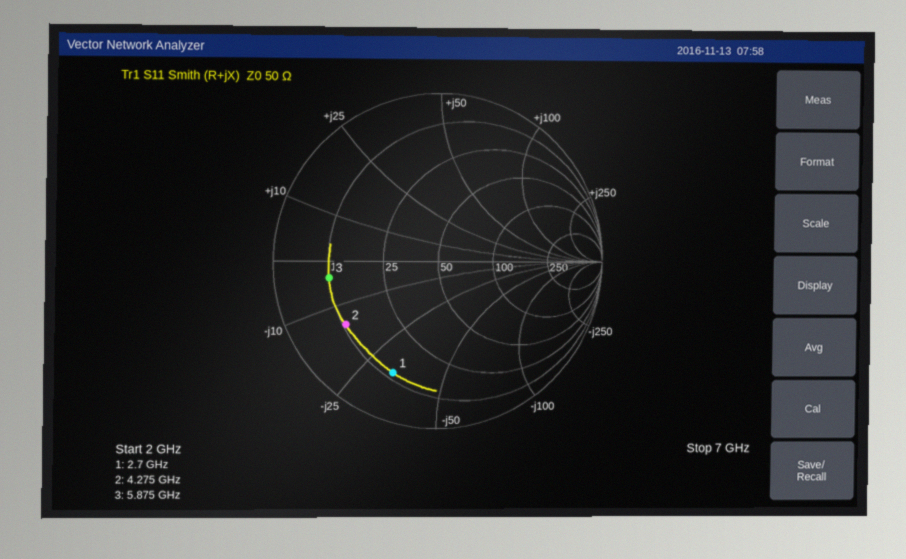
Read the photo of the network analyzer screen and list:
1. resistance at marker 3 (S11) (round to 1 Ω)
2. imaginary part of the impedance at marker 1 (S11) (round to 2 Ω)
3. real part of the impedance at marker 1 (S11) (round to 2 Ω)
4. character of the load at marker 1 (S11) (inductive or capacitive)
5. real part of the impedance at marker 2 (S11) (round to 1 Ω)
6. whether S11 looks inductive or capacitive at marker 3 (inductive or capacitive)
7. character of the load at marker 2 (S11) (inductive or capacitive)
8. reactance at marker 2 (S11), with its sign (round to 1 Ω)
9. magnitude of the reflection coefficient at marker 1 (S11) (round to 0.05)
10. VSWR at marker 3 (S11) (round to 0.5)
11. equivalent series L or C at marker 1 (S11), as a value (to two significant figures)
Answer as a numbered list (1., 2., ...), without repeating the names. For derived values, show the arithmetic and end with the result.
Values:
1. 10 Ω
2. -32 Ω
3. 12 Ω
4. capacitive
5. 11 Ω
6. capacitive
7. capacitive
8. -15 Ω
9. 0.70
10. 5.0
11. C = 1/(2π × 2.7 GHz × 32 Ω) ≈ 1.8 pF
